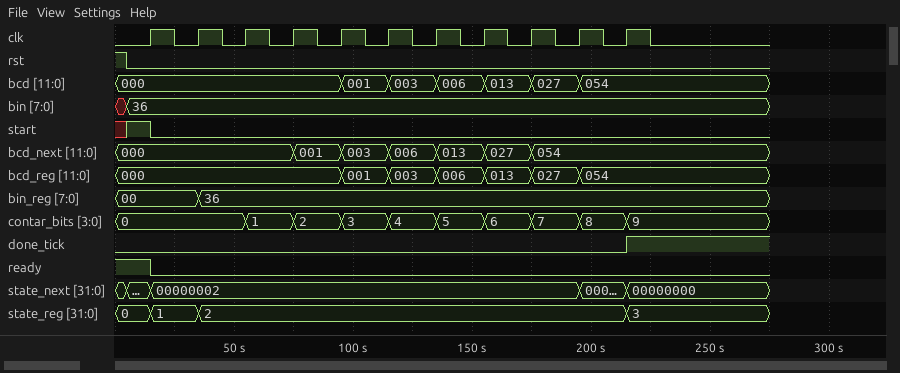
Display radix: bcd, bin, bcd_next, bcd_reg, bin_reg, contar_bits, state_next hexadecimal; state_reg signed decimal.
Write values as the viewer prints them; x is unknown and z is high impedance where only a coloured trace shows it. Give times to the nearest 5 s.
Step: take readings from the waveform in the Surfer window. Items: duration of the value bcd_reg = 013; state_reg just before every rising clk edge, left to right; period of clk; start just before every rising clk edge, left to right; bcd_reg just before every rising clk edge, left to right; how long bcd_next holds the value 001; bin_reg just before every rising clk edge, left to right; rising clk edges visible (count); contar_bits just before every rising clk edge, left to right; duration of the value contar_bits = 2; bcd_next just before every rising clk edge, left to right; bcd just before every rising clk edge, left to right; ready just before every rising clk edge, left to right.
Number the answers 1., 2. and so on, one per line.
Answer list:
1. 20 s
2. 0, 1, 2, 2, 2, 2, 2, 2, 2, 2, 2
3. 20 s
4. 1 0 0 0 0 0 0 0 0 0 0
5. 000, 000, 000, 000, 000, 001, 003, 006, 013, 027, 054
6. 20 s
7. 00, 00, 36, 36, 36, 36, 36, 36, 36, 36, 36
8. 11
9. 0, 0, 0, 1, 2, 3, 4, 5, 6, 7, 8
10. 20 s
11. 000, 000, 000, 000, 001, 003, 006, 013, 027, 054, 054
12. 000, 000, 000, 000, 000, 001, 003, 006, 013, 027, 054
13. 1 0 0 0 0 0 0 0 0 0 0
